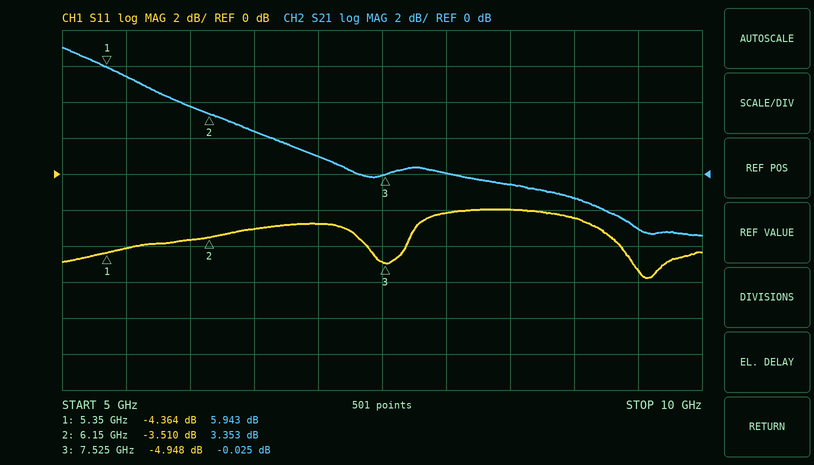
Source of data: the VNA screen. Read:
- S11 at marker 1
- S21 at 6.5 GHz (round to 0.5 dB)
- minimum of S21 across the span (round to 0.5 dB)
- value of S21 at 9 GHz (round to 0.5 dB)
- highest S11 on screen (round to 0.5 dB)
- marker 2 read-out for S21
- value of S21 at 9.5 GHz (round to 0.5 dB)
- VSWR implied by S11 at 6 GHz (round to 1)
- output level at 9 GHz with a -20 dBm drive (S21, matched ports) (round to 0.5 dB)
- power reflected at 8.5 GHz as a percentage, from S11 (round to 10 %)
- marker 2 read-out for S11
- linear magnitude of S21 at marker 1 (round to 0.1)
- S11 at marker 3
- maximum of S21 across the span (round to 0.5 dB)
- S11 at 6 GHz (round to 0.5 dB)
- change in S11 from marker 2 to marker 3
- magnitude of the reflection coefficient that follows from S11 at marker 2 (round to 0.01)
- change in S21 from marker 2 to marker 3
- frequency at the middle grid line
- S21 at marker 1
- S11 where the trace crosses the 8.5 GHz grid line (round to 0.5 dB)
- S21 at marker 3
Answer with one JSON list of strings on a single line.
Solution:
["-4.364 dB", "2.5 dB", "-3.5 dB", "-1.5 dB", "-2.0 dB", "3.353 dB", "-3.0 dB", "5", "-21.5 dBm", "60 %", "-3.510 dB", "2.0", "-4.948 dB", "7.0 dB", "-3.5 dB", "-1.438 dB", "0.67", "-3.378 dB", "7.5 GHz", "5.943 dB", "-2.0 dB", "-0.025 dB"]
